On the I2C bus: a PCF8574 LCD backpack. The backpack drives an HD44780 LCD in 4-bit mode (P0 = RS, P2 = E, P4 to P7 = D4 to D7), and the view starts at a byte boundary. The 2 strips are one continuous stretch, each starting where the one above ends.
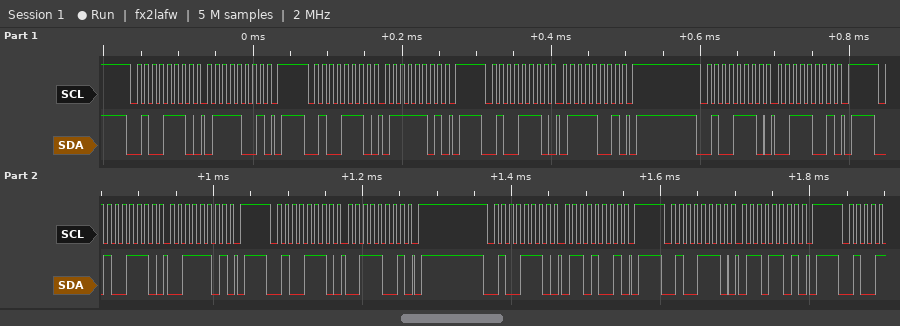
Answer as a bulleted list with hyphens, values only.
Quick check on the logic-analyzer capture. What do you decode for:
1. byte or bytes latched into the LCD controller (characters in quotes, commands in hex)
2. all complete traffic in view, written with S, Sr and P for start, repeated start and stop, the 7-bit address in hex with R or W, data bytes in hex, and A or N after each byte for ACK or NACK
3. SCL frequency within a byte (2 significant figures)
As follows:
- 's'
- S 27W A 79 A P S 27W A 7D A P S 27W A 79 A P S 27W A 39 A P S 27W A 3D A P S 27W A 39 A P S 27W A 69 A P S 27W A 6D A P
- 100 kHz
